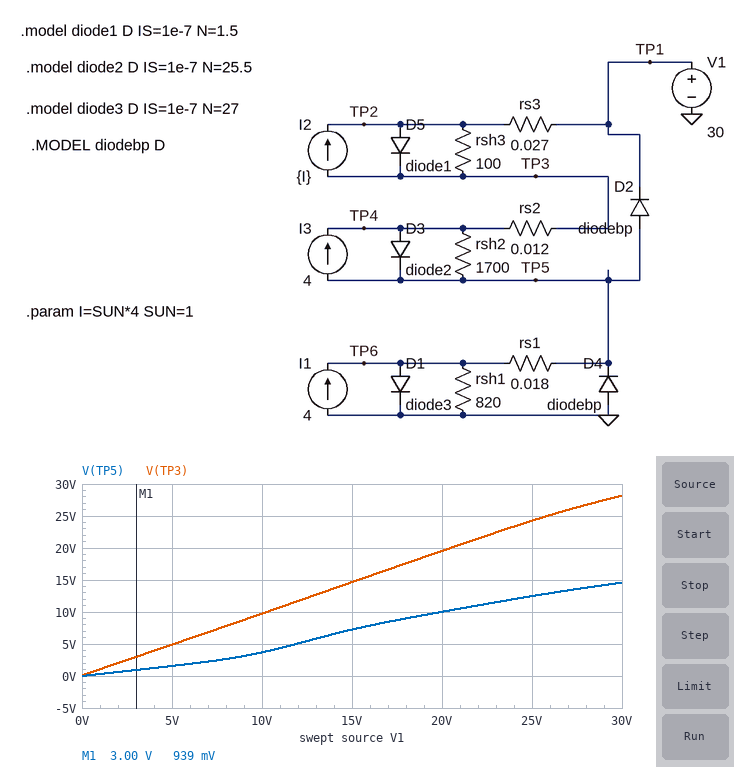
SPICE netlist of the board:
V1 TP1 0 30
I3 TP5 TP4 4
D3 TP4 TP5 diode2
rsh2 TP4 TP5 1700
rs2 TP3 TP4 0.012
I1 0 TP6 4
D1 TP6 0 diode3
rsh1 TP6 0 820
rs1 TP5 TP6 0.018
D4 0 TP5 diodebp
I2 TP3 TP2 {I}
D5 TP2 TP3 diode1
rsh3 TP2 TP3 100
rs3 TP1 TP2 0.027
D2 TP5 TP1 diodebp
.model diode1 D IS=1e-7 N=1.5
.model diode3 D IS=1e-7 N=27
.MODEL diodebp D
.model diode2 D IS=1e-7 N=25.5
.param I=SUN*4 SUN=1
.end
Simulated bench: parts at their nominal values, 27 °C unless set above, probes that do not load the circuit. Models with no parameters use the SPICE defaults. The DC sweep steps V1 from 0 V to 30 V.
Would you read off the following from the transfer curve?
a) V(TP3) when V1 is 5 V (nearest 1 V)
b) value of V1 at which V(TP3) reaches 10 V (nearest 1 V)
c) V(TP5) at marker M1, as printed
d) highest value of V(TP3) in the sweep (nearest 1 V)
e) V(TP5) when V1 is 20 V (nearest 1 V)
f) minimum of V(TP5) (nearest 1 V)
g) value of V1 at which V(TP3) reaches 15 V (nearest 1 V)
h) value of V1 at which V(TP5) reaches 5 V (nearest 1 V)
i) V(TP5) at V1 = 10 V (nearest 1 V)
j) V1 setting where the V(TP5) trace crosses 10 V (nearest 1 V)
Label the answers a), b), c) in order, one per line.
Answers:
a) 5 V
b) 10 V
c) 939 mV
d) 28 V
e) 10 V
f) 0 V
g) 15 V
h) 12 V
i) 4 V
j) 20 V
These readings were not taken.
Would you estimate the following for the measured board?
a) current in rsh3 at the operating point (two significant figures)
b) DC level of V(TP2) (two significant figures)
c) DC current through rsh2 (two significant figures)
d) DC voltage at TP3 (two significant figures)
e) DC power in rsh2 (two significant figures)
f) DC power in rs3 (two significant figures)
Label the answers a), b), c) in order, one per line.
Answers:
a) 7.7 mA
b) 29 V
c) 7.7 mA
d) 28 V
e) 100 mW
f) 41 W
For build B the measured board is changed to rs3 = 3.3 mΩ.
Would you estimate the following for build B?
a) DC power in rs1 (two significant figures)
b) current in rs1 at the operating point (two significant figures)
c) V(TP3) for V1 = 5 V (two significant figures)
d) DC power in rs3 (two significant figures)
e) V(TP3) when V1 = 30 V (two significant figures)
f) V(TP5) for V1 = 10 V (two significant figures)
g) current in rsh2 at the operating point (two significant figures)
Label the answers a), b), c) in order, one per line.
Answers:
a) 53 W
b) 54 A
c) 4.8 V
d) 9.7 W
e) 29 V
f) 3.6 V
g) 7.8 mA
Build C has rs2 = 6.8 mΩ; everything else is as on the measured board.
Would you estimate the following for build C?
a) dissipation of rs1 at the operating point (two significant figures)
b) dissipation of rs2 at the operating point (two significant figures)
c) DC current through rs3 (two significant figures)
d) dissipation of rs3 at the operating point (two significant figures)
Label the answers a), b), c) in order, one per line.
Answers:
a) 31 W
b) 12 W
c) 42 A
d) 47 W
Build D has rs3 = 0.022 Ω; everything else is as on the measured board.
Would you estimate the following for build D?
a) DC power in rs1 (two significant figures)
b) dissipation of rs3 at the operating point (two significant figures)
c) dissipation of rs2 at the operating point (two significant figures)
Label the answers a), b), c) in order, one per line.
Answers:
a) 31 W
b) 38 W
c) 21 W
